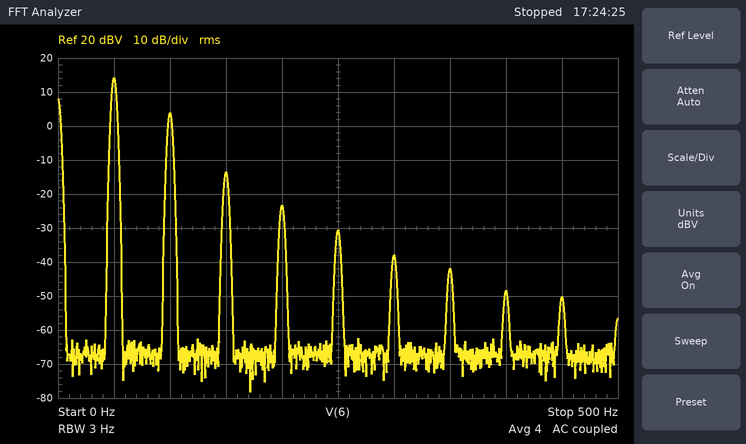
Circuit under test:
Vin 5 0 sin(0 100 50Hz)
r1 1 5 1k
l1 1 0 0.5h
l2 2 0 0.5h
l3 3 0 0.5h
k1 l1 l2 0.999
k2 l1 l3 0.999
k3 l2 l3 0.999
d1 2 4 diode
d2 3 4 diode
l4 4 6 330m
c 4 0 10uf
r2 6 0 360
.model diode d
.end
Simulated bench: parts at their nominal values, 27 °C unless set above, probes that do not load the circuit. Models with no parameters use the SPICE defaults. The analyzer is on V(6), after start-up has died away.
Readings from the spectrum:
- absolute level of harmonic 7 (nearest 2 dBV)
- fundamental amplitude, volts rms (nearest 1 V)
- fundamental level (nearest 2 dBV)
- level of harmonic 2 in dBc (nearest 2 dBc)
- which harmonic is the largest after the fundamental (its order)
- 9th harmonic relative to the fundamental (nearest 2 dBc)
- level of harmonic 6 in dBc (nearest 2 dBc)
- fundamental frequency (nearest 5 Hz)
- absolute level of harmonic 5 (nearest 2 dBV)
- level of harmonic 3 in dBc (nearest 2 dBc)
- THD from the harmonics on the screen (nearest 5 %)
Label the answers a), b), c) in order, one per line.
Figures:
a) -42 dBV
b) 5 V
c) 14 dBV
d) -10 dBc
e) 2
f) -64 dBc
g) -52 dBc
h) 50 Hz
i) -30 dBV
j) -28 dBc
k) 30 %
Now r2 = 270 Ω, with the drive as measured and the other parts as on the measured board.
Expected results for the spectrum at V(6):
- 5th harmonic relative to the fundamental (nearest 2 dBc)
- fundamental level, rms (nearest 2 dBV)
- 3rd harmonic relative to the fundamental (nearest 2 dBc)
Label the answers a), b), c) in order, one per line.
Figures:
a) -50 dBc
b) 14 dBV
c) -32 dBc
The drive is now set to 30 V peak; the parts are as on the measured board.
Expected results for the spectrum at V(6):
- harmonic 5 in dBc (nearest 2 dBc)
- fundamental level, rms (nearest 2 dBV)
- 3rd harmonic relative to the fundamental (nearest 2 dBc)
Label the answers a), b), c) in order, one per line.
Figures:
a) -42 dBc
b) 2 dBV
c) -26 dBc
